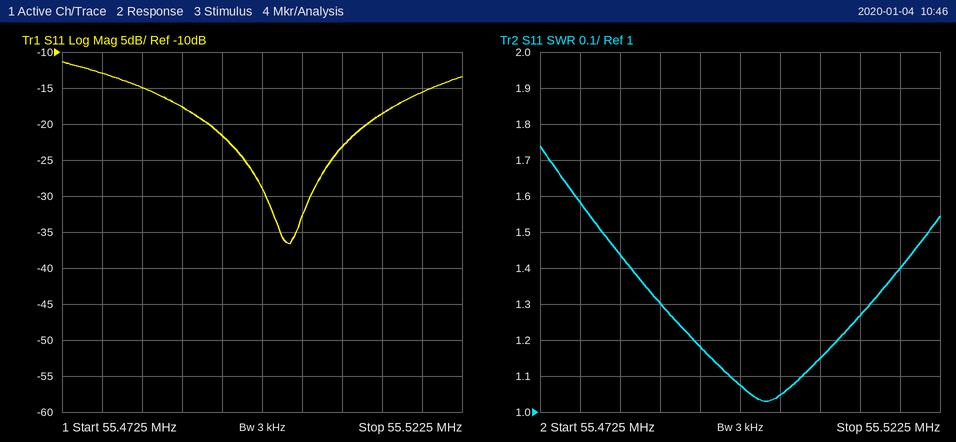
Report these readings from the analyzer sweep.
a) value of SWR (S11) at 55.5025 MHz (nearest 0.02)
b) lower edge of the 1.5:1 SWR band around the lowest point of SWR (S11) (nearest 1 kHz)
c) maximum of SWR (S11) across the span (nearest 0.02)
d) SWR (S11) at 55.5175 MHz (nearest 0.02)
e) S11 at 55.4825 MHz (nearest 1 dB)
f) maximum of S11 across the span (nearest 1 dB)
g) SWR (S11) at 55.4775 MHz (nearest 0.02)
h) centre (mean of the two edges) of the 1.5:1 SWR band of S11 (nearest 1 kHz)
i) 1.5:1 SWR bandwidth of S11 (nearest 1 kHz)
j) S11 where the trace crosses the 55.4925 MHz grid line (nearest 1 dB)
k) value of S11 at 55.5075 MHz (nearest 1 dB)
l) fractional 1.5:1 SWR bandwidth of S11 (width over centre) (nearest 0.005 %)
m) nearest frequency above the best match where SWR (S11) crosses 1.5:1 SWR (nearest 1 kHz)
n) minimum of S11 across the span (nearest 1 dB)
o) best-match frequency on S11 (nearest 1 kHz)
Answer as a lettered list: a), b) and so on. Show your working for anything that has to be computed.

a) 1.04
b) 55.480 MHz
c) 1.74
d) 1.40
e) -15 dB
f) -11 dB
g) 1.58
h) 55.501 MHz
i) 55.521 MHz − 55.480 MHz = 41 kHz
j) -22 dB
k) -23 dB
l) 41 kHz / 55.5005 MHz ≈ 0.0739 %, so 0.075 % to the nearest 0.005 %
m) 55.521 MHz
n) -37 dB
o) 55.501 MHz
